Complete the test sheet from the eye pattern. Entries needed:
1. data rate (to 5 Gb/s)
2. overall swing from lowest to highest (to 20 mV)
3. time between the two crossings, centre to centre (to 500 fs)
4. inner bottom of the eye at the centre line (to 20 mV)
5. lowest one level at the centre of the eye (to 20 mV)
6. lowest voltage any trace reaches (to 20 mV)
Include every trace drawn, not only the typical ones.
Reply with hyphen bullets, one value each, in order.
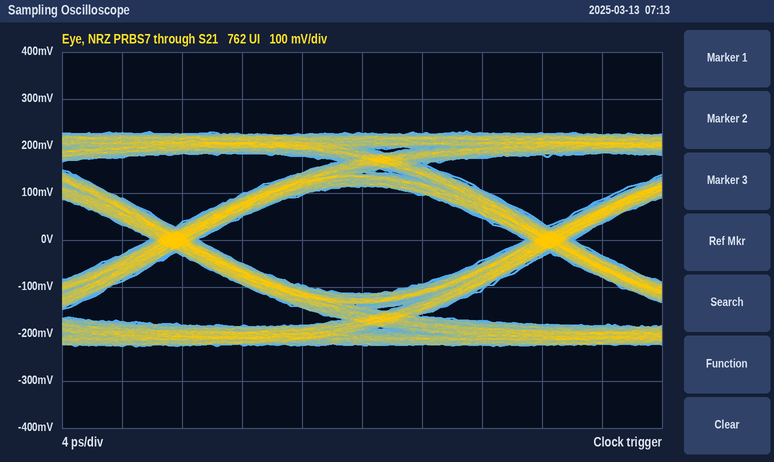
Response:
- 40 Gb/s
- 460 mV
- 25.0 ps
- -120 mV
- 120 mV
- -220 mV
